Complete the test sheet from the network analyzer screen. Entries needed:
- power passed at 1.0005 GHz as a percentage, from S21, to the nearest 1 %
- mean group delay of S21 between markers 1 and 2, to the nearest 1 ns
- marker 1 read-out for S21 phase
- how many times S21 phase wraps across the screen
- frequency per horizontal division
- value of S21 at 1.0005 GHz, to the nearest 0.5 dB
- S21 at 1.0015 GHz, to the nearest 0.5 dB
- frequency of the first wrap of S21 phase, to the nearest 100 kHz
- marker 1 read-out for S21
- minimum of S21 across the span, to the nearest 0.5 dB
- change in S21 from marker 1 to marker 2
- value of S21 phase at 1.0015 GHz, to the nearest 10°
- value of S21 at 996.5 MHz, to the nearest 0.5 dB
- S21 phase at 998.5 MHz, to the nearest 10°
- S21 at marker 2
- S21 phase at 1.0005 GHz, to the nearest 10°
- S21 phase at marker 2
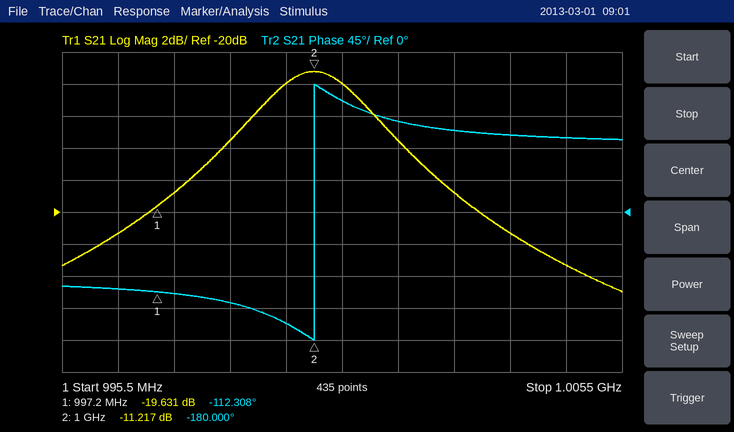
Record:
6 %
67 ns
-112.308°
1
1 MHz
-12.0 dB
-15.5 dB
1.0000 GHz
-19.631 dB
-25.0 dB
8.414 dB
130°
-21.5 dB
-130°
-11.217 dB
160°
-180.000°
